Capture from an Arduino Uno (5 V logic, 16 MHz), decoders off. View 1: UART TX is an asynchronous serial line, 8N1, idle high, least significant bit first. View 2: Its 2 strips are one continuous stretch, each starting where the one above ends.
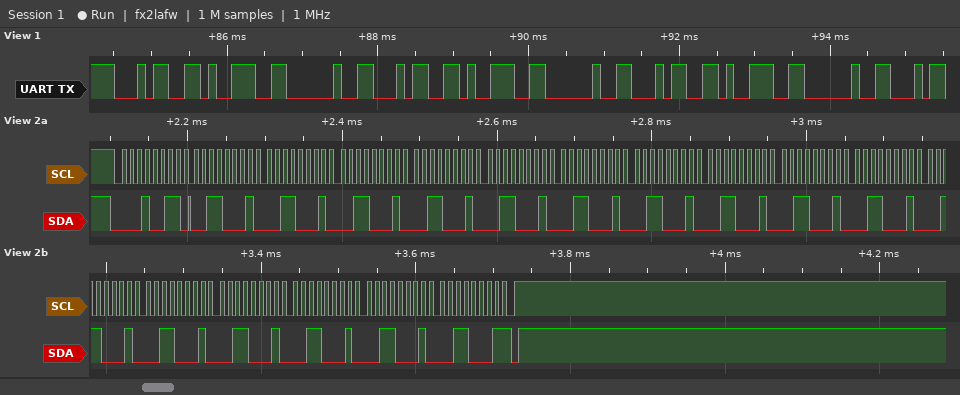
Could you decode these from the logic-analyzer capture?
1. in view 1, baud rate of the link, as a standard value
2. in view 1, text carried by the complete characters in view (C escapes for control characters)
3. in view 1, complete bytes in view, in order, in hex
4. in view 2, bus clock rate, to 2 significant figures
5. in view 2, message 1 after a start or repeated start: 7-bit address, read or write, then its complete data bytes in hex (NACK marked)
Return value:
9600 baud
"49 49 49 "
34 39 20 34 39 20 34 39 20
100 kHz
0x09 read: 31 31 31 31 31 31 31 31 31 31 31 31 31 31 31 31 NACK
